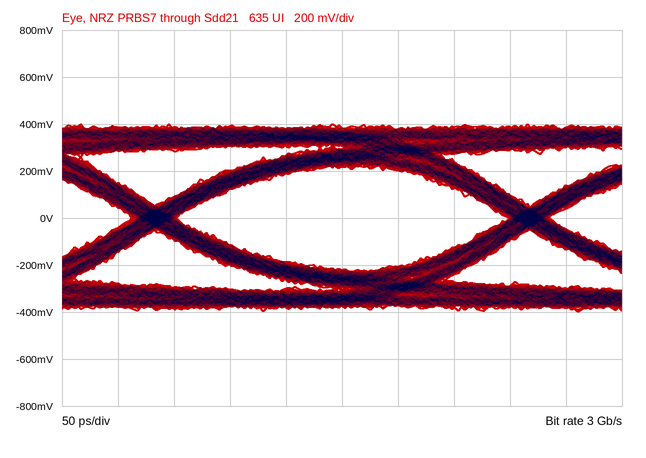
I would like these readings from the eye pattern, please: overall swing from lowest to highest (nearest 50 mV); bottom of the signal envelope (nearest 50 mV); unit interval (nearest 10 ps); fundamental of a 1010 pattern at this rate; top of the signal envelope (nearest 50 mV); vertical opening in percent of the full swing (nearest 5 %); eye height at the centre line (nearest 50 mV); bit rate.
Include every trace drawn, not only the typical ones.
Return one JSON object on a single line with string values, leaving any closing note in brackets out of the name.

{"overall swing from lowest to highest": "800 mV", "bottom of the signal envelope": "-400 mV", "unit interval": "330 ps", "fundamental of a 1010 pattern at this rate": "1.5 GHz", "top of the signal envelope": "400 mV", "vertical opening in percent of the full swing": "55 %", "eye height at the centre line": "450 mV", "bit rate": "3 Gb/s"}
